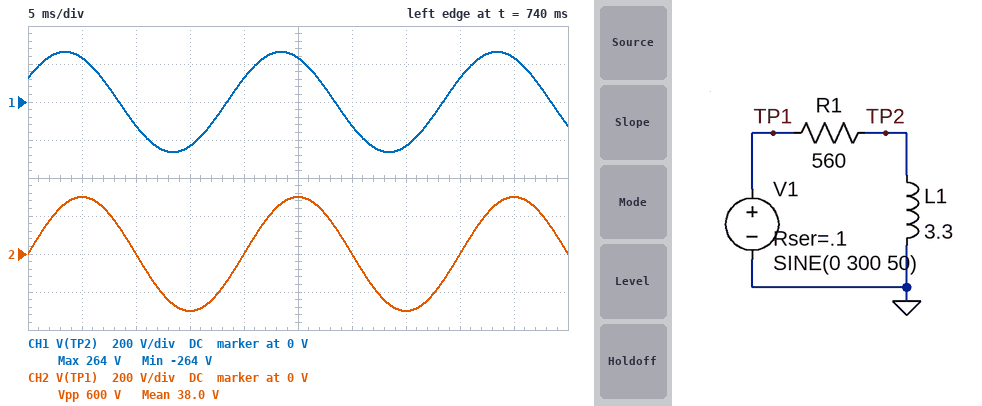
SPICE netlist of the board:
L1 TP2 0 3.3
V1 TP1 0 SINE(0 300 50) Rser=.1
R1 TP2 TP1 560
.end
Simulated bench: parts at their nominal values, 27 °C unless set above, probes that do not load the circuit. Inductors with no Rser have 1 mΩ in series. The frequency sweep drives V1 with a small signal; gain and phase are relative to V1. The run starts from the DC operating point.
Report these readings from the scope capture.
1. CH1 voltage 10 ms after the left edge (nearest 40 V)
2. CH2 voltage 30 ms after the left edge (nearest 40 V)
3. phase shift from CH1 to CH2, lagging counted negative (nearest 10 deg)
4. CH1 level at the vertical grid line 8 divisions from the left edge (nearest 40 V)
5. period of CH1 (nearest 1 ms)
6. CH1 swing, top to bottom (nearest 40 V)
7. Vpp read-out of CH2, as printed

-120 V
0 V
-30 deg
120 V
20 ms
520 V
600 V
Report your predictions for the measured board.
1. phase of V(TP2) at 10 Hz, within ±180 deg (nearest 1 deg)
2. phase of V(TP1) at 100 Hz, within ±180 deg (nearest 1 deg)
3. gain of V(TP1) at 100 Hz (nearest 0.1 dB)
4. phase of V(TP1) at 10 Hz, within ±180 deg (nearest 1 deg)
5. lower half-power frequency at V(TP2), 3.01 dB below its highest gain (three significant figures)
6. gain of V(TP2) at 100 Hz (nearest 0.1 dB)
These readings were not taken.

70 deg
0 deg
0 dB
0 deg
27.0 Hz
-0.3 dB
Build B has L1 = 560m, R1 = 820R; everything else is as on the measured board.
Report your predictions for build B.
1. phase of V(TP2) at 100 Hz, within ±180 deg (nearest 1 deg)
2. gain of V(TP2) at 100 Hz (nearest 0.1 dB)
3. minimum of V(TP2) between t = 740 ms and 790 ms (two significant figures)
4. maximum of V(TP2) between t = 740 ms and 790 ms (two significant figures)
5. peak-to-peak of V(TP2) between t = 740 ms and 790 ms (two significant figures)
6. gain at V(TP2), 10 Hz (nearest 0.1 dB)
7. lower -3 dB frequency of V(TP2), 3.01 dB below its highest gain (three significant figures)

67 deg
-8.1 dB
-63 V
63 V
130 V
-27.4 dB
233 Hz
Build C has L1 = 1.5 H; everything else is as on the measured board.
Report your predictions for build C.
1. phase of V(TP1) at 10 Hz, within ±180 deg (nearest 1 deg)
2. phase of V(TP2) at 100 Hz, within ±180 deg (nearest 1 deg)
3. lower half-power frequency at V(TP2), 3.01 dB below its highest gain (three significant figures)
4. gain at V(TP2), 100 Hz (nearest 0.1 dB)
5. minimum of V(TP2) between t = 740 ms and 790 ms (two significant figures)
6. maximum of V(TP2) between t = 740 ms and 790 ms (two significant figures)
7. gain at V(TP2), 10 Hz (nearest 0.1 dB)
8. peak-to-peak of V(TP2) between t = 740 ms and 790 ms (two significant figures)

0 deg
31 deg
59.4 Hz
-1.3 dB
-190 V
190 V
-15.6 dB
390 V
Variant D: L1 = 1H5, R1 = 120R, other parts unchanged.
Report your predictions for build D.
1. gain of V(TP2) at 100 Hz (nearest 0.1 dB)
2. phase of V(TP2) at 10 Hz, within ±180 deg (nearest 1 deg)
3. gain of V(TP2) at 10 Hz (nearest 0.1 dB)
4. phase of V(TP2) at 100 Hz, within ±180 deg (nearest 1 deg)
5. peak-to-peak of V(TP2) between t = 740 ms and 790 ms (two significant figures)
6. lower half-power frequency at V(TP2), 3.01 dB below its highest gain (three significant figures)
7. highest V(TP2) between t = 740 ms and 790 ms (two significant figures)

-0.1 dB
52 deg
-4.2 dB
7 deg
580 V
12.7 Hz
290 V
